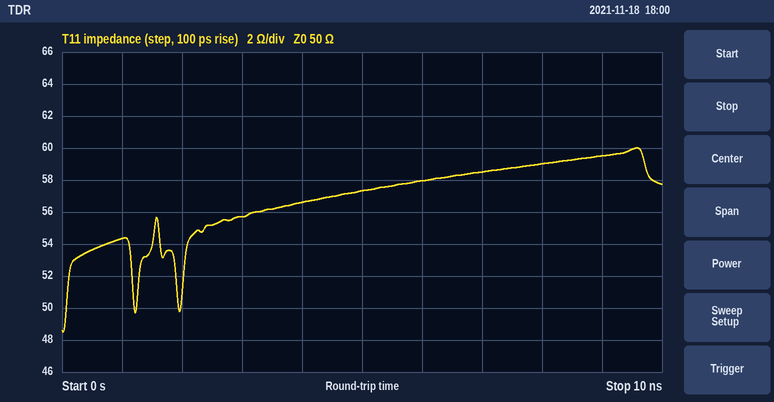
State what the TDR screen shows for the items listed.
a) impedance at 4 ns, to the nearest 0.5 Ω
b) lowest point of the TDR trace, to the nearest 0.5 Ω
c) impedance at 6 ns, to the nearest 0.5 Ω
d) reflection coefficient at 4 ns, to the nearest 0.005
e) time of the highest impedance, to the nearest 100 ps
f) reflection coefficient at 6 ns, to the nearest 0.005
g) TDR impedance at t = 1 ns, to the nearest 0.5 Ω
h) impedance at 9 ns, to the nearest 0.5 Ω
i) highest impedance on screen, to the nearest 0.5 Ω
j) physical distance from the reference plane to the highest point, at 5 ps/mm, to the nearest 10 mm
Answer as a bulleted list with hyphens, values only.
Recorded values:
- 56.5 Ω
- 48.5 Ω
- 58.0 Ω
- +0.060
- 9.6 ns
- +0.075
- 54.5 Ω
- 59.5 Ω
- 60.0 Ω
- 960 mm
